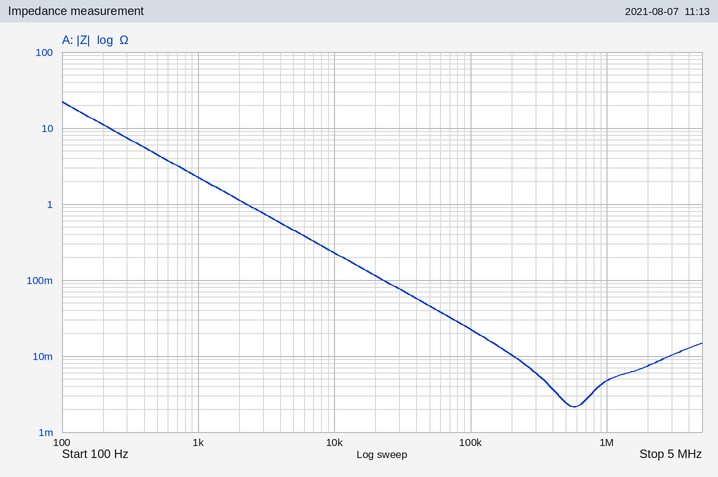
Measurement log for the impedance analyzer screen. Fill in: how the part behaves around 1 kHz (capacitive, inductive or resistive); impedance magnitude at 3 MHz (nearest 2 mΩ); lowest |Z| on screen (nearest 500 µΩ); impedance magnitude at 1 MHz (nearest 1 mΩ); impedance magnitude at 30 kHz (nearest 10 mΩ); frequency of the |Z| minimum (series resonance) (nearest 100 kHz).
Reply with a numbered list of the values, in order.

1. capacitive
2. 10 mΩ
3. 2.0 mΩ
4. 5 mΩ
5. 80 mΩ
6. 600 kHz
